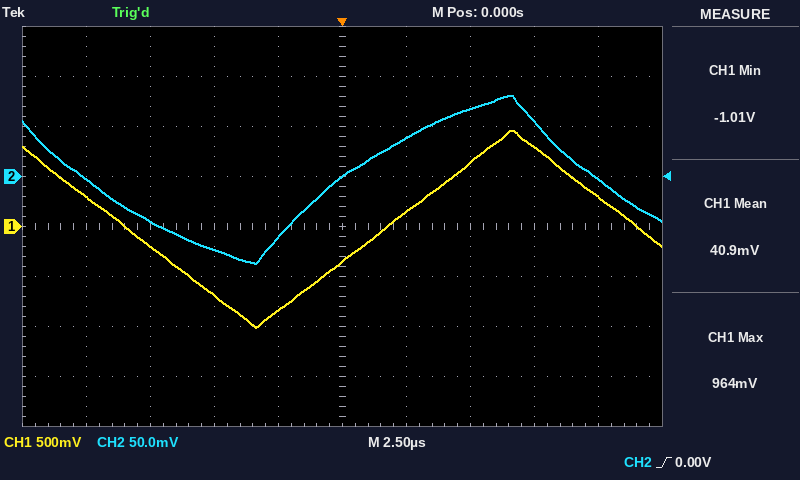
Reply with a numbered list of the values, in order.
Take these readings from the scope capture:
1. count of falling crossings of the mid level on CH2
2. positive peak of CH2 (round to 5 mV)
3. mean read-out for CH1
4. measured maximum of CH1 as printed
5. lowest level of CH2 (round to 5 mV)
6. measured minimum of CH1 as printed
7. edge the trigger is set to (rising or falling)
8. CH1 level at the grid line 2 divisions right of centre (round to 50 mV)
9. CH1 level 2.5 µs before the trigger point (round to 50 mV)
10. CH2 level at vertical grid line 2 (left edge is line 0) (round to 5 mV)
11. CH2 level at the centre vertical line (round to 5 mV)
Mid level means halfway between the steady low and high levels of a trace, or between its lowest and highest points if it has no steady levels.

1. 2
2. 80 mV
3. 40.9 mV
4. 964 mV
5. -85 mV
6. -1.01 V
7. rising
8. 650 mV
9. -850 mV
10. -45 mV
11. 0 mV
